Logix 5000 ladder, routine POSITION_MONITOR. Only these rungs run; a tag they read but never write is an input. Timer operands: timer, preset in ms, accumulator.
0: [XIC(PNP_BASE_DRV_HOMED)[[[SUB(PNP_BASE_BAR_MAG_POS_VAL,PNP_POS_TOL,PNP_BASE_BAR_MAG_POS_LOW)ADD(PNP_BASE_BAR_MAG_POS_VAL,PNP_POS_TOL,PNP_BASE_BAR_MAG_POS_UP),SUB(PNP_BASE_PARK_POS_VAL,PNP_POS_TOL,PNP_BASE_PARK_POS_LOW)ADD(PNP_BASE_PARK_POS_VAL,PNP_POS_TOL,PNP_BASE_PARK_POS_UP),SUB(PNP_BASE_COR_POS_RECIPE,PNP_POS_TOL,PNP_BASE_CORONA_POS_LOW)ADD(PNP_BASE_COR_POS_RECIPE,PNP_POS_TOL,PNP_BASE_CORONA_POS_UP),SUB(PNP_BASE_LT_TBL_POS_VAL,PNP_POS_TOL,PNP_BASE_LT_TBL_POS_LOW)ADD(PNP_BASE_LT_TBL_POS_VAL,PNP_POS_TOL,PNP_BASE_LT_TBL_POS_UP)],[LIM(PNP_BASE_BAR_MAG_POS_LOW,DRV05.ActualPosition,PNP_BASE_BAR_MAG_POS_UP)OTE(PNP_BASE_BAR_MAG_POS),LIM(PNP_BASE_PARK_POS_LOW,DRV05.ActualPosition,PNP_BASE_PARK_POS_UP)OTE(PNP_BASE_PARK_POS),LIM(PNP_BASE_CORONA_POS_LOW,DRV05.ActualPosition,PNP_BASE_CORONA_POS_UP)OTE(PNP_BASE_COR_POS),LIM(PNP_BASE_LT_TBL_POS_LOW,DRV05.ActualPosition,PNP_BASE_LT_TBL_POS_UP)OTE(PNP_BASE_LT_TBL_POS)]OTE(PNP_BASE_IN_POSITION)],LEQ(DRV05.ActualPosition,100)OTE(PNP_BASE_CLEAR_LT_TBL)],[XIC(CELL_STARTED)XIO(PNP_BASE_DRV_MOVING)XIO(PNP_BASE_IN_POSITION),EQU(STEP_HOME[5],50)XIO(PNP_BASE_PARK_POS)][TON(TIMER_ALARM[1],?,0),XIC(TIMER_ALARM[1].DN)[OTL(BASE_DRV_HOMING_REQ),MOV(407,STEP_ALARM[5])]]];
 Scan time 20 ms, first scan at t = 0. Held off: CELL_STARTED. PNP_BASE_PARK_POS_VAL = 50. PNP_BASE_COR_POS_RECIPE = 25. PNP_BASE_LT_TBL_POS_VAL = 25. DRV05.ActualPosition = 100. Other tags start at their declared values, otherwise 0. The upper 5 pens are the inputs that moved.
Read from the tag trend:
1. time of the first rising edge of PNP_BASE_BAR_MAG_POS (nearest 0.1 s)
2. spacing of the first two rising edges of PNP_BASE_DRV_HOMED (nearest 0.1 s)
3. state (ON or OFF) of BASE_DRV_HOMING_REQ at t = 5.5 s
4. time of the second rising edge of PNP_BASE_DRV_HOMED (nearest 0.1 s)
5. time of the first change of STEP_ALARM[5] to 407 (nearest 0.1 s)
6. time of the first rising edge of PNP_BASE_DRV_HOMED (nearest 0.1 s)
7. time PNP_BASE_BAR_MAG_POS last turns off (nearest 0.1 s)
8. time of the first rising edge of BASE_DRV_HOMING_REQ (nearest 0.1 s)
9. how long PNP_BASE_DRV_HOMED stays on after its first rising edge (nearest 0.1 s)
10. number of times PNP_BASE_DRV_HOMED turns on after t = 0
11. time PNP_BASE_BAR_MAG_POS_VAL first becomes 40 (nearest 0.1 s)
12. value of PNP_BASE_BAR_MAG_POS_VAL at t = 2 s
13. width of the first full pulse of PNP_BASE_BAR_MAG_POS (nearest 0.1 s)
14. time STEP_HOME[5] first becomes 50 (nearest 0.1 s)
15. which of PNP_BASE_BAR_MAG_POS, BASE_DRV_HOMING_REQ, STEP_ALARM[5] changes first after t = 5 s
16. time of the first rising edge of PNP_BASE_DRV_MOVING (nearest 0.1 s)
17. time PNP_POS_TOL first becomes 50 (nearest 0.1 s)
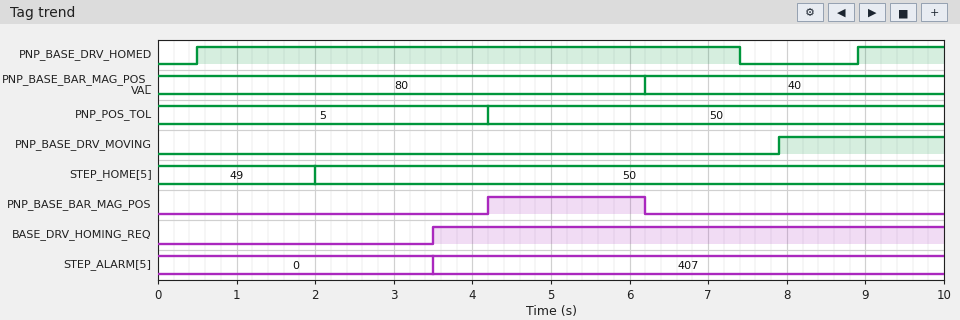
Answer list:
4.2 s
8.4 s
ON
8.9 s
3.5 s
0.5 s
6.2 s
3.5 s
6.9 s
2
6.2 s
80
2.0 s
2.0 s
PNP_BASE_BAR_MAG_POS
7.9 s
4.2 s
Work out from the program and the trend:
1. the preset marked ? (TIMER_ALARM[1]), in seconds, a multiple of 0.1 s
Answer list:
1.5 s
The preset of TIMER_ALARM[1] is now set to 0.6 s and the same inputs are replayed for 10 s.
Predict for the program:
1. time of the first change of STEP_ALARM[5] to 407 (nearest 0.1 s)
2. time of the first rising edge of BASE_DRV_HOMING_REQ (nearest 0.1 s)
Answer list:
2.6 s
2.6 s
